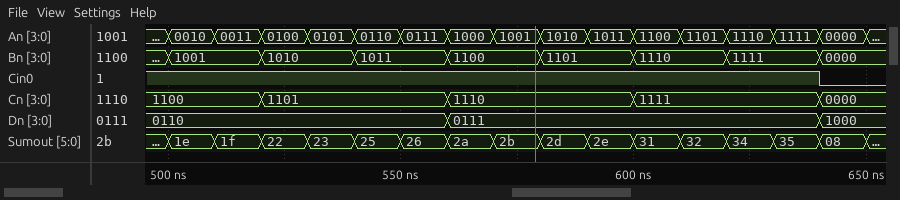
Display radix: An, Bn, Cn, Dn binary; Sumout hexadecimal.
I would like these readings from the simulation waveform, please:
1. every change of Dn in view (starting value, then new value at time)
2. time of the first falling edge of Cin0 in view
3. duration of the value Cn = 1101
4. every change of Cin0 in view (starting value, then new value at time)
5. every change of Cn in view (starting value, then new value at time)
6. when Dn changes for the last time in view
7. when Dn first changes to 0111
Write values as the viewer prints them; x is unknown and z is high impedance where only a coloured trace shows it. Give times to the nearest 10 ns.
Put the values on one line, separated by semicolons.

0110, 0111 at 560 ns, 1000 at 640 ns; 640 ns; 40 ns; 1, 0 at 640 ns; 1100, 1101 at 520 ns, 1110 at 560 ns, 1111 at 600 ns, 0000 at 640 ns; 640 ns; 560 ns
